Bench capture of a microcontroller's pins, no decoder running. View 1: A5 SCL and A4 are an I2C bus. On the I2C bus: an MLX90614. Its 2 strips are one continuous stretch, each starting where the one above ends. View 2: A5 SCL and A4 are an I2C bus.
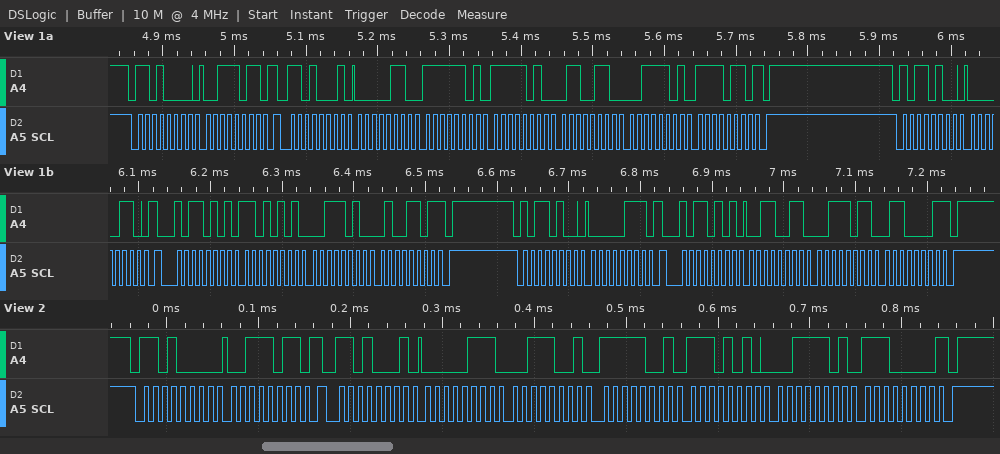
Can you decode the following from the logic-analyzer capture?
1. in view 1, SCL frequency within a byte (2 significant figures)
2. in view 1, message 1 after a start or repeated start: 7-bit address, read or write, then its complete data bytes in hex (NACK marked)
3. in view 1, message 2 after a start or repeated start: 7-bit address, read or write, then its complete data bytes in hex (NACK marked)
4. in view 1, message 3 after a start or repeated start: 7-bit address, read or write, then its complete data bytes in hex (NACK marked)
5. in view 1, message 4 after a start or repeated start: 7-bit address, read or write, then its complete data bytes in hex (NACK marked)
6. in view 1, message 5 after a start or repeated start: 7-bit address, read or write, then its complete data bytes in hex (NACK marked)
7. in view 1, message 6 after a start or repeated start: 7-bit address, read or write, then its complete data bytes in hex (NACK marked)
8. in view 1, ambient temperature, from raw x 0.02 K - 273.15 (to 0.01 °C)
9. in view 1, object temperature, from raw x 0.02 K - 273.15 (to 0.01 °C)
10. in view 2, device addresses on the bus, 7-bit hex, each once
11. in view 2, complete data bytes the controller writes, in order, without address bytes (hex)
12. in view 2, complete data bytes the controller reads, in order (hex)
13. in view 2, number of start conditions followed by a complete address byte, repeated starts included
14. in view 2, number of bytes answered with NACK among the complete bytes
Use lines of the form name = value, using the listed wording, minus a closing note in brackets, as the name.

in view 1, SCL frequency within a byte = 100 kHz
in view 1, message 1 after a start or repeated start: 7-bit address, read or write, then its complete data bytes in hex = 0x68 write: 3B
in view 1, message 2 after a start or repeated start: 7-bit address, read or write, then its complete data bytes in hex = 0x68 read: 06 FD FA 66 3D F6 NACK
in view 1, message 3 after a start or repeated start: 7-bit address, read or write, then its complete data bytes in hex = 0x5A write: 06
in view 1, message 4 after a start or repeated start: 7-bit address, read or write, then its complete data bytes in hex = 0x5A read: D5 3A 4D NACK
in view 1, message 5 after a start or repeated start: 7-bit address, read or write, then its complete data bytes in hex = 0x5A write: 07
in view 1, message 6 after a start or repeated start: 7-bit address, read or write, then its complete data bytes in hex = 0x5A read: 33 3B 61 NACK
in view 1, ambient temperature, from raw x 0.02 K - 273.15 = 28.07 °C
in view 1, object temperature, from raw x 0.02 K - 273.15 = 29.95 °C
in view 2, device addresses on the bus, 7-bit hex, each once = 0x68
in view 2, complete data bytes the controller writes, in order, without address bytes = 3B
in view 2, complete data bytes the controller reads, in order = 07 39 F9 EA 3D E0
in view 2, number of start conditions followed by a complete address byte, repeated starts included = 2
in view 2, number of bytes answered with NACK among the complete bytes = 1
